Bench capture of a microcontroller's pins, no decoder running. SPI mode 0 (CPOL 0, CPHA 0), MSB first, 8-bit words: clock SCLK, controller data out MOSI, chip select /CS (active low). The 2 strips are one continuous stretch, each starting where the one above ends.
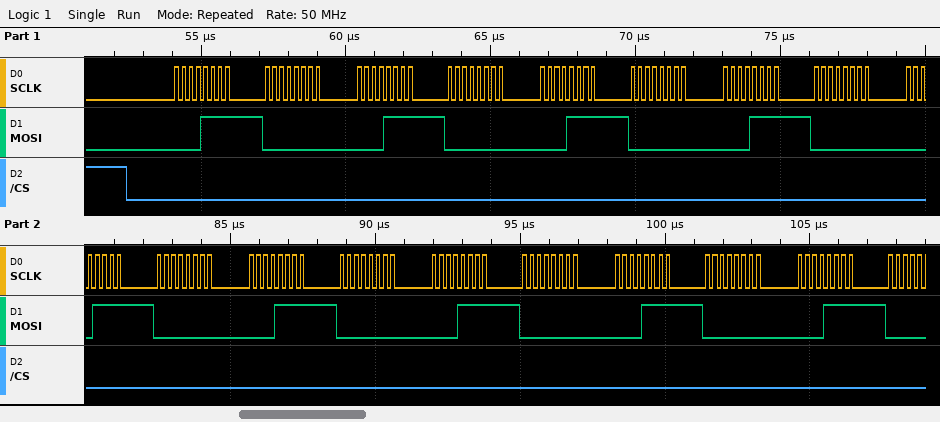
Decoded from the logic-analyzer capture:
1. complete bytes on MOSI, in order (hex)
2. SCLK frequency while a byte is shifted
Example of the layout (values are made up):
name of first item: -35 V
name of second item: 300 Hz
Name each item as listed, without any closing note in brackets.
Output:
complete bytes on MOSI, in order: 0x0F 0x00 0x0F 0x00 0x0F 0x00 0x0F 0x00 0x0F 0x00 0x0F 0x00 0x0F 0x00 0x0F 0x00 0x0F
SCLK frequency while a byte is shifted: 4 MHz
